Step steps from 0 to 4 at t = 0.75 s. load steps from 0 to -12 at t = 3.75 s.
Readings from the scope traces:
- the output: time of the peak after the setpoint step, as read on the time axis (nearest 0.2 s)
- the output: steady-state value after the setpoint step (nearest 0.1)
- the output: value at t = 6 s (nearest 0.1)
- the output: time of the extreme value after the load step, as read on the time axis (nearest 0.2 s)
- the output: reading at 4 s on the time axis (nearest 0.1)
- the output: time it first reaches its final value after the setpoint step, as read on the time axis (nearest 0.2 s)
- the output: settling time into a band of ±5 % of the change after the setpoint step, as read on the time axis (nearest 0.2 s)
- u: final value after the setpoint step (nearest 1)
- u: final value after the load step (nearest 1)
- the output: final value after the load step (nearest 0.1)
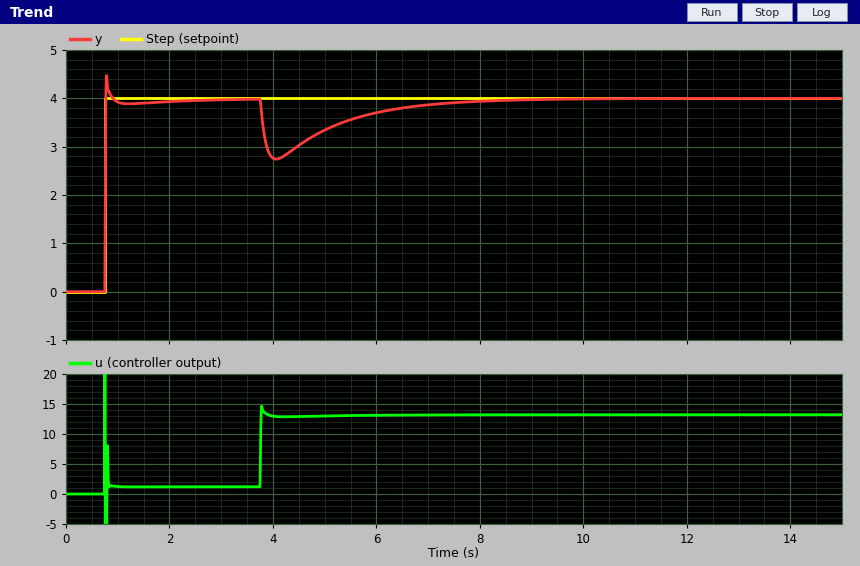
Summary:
0.8 s
4.0
3.7
4.0 s
2.8
0.8 s
0.8 s
1
13
4.0
